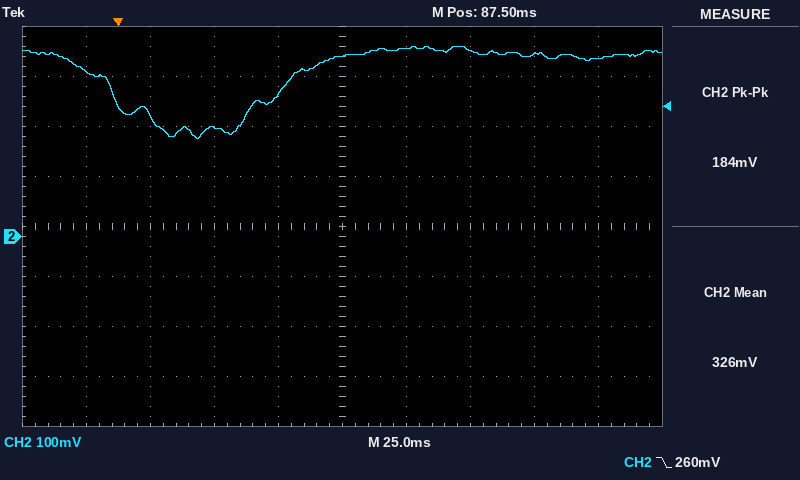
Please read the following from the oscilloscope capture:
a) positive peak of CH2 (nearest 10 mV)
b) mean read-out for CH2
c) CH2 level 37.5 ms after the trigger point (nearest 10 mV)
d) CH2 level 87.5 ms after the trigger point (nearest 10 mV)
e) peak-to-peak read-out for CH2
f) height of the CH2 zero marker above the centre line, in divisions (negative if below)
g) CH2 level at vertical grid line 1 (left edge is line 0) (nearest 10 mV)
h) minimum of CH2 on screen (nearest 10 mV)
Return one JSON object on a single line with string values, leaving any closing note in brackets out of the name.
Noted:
{"positive peak of CH2": "380 mV", "mean read-out for CH2": "326 mV", "CH2 level 37.5 ms after the trigger point": "220 mV", "CH2 level 87.5 ms after the trigger point": "360 mV", "peak-to-peak read-out for CH2": "184 mV", "height of the CH2 zero marker above the centre line, in divisions": "-0.2 div", "CH2 level at vertical grid line 1 (left edge is line 0)": "330 mV", "minimum of CH2 on screen": "200 mV"}
